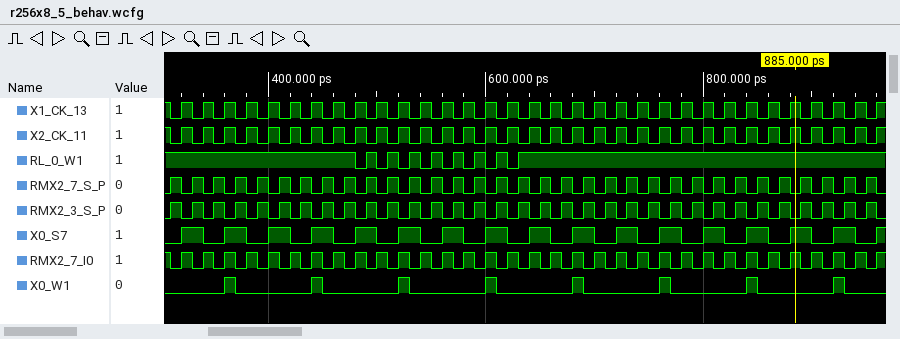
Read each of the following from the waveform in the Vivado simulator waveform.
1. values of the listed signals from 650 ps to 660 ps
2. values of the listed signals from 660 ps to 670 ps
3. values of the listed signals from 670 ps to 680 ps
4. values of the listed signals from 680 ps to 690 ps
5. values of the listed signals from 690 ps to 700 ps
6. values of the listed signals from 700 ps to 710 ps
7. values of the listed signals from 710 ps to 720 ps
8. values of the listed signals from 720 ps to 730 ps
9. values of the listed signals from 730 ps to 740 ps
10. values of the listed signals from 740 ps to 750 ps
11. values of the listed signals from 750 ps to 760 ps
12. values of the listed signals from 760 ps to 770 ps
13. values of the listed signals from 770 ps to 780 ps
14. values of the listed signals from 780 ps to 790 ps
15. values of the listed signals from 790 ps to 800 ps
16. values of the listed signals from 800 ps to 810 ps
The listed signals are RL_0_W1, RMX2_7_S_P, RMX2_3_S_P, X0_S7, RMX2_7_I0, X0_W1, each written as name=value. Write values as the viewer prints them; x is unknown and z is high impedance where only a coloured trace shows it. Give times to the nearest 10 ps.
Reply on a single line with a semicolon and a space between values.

RL_0_W1=1, RMX2_7_S_P=1, RMX2_3_S_P=1, X0_S7=1, RMX2_7_I0=0, X0_W1=0; RL_0_W1=1, RMX2_7_S_P=0, RMX2_3_S_P=0, X0_S7=0, RMX2_7_I0=1, X0_W1=0; RL_0_W1=1, RMX2_7_S_P=1, RMX2_3_S_P=1, X0_S7=0, RMX2_7_I0=0, X0_W1=0; RL_0_W1=1, RMX2_7_S_P=0, RMX2_3_S_P=0, X0_S7=1, RMX2_7_I0=1, X0_W1=1; RL_0_W1=1, RMX2_7_S_P=1, RMX2_3_S_P=1, X0_S7=1, RMX2_7_I0=0, X0_W1=0; RL_0_W1=1, RMX2_7_S_P=0, RMX2_3_S_P=0, X0_S7=0, RMX2_7_I0=1, X0_W1=0; RL_0_W1=1, RMX2_7_S_P=1, RMX2_3_S_P=1, X0_S7=0, RMX2_7_I0=0, X0_W1=0; RL_0_W1=1, RMX2_7_S_P=0, RMX2_3_S_P=0, X0_S7=1, RMX2_7_I0=1, X0_W1=0; RL_0_W1=1, RMX2_7_S_P=1, RMX2_3_S_P=1, X0_S7=1, RMX2_7_I0=0, X0_W1=0; RL_0_W1=1, RMX2_7_S_P=0, RMX2_3_S_P=0, X0_S7=0, RMX2_7_I0=1, X0_W1=0; RL_0_W1=1, RMX2_7_S_P=1, RMX2_3_S_P=1, X0_S7=0, RMX2_7_I0=0, X0_W1=0; RL_0_W1=1, RMX2_7_S_P=0, RMX2_3_S_P=0, X0_S7=1, RMX2_7_I0=1, X0_W1=1; RL_0_W1=1, RMX2_7_S_P=1, RMX2_3_S_P=1, X0_S7=1, RMX2_7_I0=0, X0_W1=0; RL_0_W1=1, RMX2_7_S_P=0, RMX2_3_S_P=0, X0_S7=0, RMX2_7_I0=1, X0_W1=0; RL_0_W1=1, RMX2_7_S_P=1, RMX2_3_S_P=1, X0_S7=0, RMX2_7_I0=0, X0_W1=0; RL_0_W1=1, RMX2_7_S_P=0, RMX2_3_S_P=0, X0_S7=1, RMX2_7_I0=1, X0_W1=0
